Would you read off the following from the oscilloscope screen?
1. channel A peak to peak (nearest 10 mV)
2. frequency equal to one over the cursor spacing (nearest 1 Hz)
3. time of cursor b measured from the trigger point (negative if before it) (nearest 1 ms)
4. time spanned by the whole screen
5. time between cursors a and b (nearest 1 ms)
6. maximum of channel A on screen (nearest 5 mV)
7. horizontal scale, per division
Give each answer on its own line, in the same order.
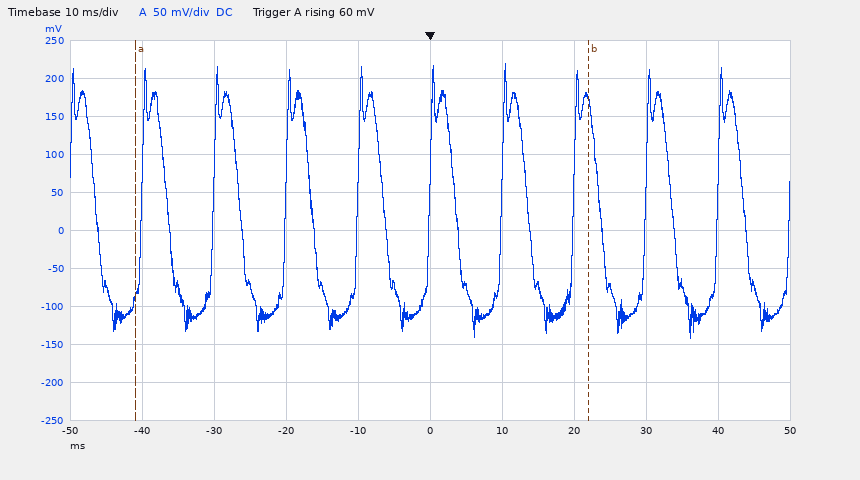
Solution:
360 mV
16 Hz
+22 ms
100 ms
63 ms
220 mV
10 ms
